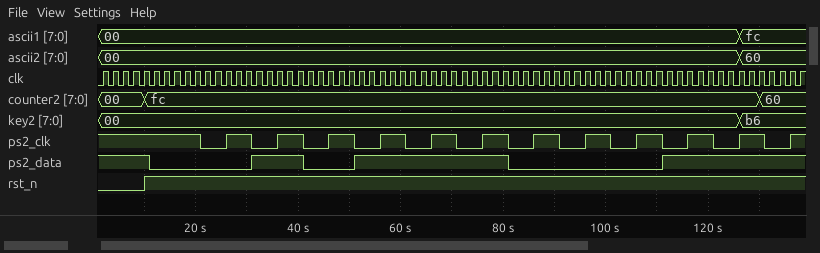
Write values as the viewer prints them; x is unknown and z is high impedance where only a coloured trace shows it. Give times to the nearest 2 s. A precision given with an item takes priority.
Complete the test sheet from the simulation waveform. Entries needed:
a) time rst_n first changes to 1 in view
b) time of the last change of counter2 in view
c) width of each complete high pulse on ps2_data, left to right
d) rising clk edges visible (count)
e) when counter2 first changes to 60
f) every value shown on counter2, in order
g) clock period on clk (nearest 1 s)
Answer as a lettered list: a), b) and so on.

a) 10 s
b) 130 s
c) 10 s, 30 s
d) 69
e) 130 s
f) 00, fc, 60
g) 2 s
